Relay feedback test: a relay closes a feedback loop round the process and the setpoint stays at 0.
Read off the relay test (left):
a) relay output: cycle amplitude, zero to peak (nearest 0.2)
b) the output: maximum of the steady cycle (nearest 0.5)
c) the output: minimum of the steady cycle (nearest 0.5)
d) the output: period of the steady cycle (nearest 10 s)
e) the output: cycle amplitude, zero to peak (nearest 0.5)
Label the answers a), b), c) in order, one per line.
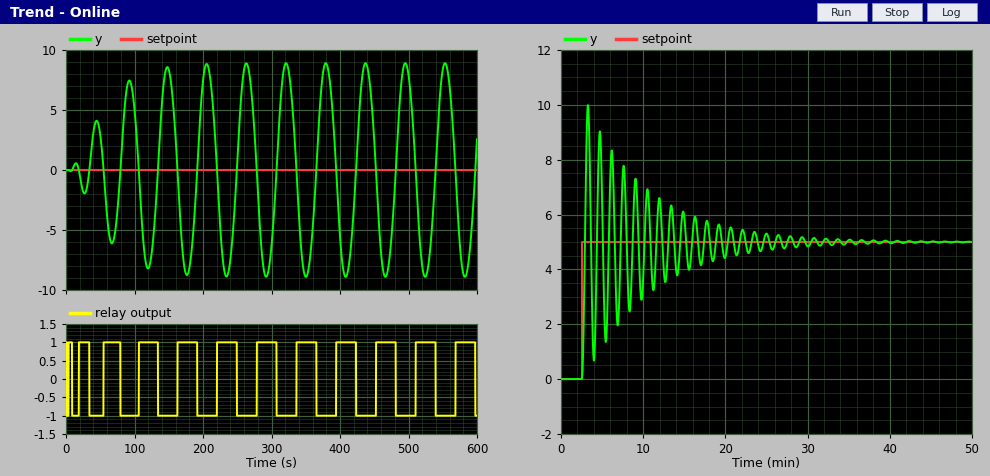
a) 1.0
b) 9.0
c) -9.0
d) 60 s
e) 9.0
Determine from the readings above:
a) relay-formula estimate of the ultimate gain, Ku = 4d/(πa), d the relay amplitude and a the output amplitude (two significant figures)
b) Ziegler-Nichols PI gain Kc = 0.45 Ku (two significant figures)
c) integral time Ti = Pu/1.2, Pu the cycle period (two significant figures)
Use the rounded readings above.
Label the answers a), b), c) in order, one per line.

a) 0.14
b) 0.063
c) 50 s
